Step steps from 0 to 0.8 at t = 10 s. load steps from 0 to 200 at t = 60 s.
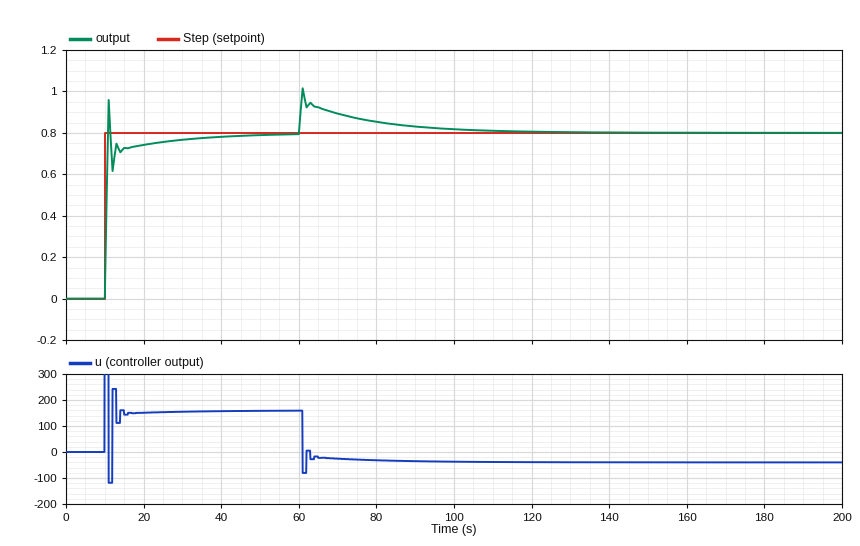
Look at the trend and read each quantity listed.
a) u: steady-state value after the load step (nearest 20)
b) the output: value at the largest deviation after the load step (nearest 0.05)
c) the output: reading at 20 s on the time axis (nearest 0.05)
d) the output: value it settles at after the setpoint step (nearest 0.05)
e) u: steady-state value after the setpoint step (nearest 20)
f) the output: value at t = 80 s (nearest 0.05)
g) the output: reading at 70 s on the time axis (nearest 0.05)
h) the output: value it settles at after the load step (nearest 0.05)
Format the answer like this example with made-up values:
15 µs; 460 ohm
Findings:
-40; 1.00; 0.75; 0.80; 160; 0.85; 0.90; 0.80
